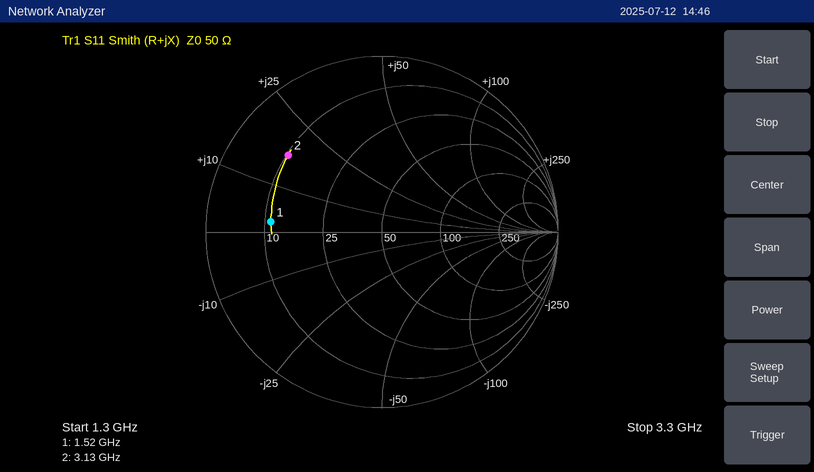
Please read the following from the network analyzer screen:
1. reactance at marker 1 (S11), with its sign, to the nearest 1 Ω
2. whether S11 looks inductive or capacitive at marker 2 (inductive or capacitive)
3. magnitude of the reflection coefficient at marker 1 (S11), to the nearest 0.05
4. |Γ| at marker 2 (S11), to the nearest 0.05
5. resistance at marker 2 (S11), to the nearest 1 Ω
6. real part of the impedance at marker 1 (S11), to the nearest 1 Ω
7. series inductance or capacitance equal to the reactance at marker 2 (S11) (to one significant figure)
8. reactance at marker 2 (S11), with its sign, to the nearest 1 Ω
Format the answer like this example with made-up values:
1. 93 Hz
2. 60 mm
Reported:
1. +2 Ω
2. inductive
3. 0.65
4. 0.70
5. 10 Ω
6. 11 Ω
7. 900 pH
8. +17 Ω
